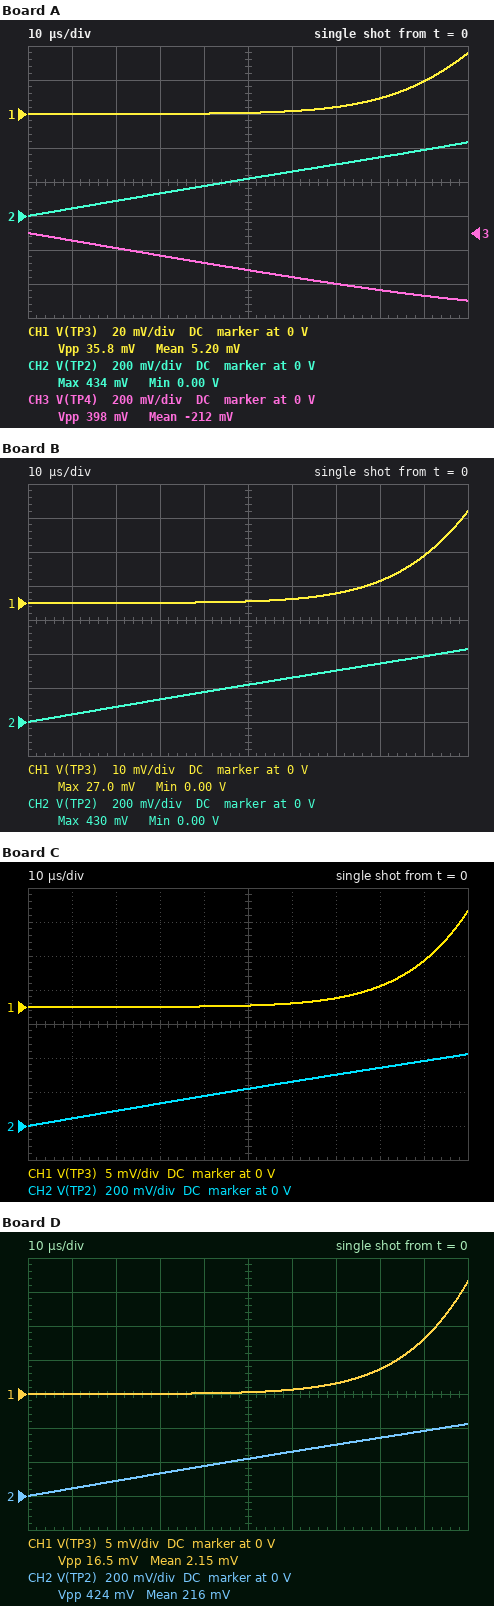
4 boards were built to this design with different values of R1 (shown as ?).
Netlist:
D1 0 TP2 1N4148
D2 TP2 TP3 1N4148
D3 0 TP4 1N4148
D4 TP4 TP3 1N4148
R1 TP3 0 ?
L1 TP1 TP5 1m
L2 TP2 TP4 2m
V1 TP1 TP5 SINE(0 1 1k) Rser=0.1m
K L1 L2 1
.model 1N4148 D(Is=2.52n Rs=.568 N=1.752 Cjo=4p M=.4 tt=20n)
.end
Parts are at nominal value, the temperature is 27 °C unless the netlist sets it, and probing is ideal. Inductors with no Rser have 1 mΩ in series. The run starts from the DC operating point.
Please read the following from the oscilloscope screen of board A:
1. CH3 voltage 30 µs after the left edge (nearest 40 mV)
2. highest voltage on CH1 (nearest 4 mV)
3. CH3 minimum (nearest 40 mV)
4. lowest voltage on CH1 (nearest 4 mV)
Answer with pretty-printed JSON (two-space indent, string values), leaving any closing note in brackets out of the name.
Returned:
{
  "CH3 voltage 30 µs after the left edge": "-120 mV",
  "highest voltage on CH1": "36 mV",
  "CH3 minimum": "-400 mV",
  "lowest voltage on CH1": "0 V"
}
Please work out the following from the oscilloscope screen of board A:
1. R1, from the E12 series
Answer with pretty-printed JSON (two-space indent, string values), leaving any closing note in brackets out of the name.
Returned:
{
  "R1, from the E12 series": "2.2 kΩ"
}
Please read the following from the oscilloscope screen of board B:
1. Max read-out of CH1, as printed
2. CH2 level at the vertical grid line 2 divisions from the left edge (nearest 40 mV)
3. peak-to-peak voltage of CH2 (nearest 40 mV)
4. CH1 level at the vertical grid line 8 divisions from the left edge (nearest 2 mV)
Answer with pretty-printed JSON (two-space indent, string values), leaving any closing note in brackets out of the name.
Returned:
{
  "Max read-out of CH1, as printed": "27.0 mV",
  "CH2 level at the vertical grid line 2 divisions from the left edge": "80 mV",
  "peak-to-peak voltage of CH2": "440 mV",
  "CH1 level at the vertical grid line 8 divisions from the left edge": "6 mV"
}
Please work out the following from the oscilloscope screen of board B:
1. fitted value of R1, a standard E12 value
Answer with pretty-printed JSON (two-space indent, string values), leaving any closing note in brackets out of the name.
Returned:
{
  "fitted value of R1, a standard E12 value": "1.5 kΩ"
}
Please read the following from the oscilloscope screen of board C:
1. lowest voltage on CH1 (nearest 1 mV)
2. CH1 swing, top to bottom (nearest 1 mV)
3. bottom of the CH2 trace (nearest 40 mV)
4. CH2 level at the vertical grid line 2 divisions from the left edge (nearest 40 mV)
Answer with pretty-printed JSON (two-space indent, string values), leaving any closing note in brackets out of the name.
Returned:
{
  "lowest voltage on CH1": "0 V",
  "CH1 swing, top to bottom": "14 mV",
  "bottom of the CH2 trace": "0 V",
  "CH2 level at the vertical grid line 2 divisions from the left edge": "80 mV"
}
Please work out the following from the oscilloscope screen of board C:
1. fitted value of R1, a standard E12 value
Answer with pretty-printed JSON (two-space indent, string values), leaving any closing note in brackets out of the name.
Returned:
{
  "fitted value of R1, a standard E12 value": "680 Ω"
}
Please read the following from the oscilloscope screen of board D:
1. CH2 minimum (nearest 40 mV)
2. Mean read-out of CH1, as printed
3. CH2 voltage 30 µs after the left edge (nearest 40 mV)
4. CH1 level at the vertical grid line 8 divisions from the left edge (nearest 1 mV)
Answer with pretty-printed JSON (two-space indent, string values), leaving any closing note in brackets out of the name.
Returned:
{
  "CH2 minimum": "0 V",
  "Mean read-out of CH1, as printed": "2.15 mV",
  "CH2 voltage 30 µs after the left edge": "120 mV",
  "CH1 level at the vertical grid line 8 divisions from the left edge": "4 mV"
}
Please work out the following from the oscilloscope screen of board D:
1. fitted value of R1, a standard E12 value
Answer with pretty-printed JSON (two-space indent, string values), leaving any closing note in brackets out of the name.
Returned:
{
  "fitted value of R1, a standard E12 value": "820 Ω"
}
